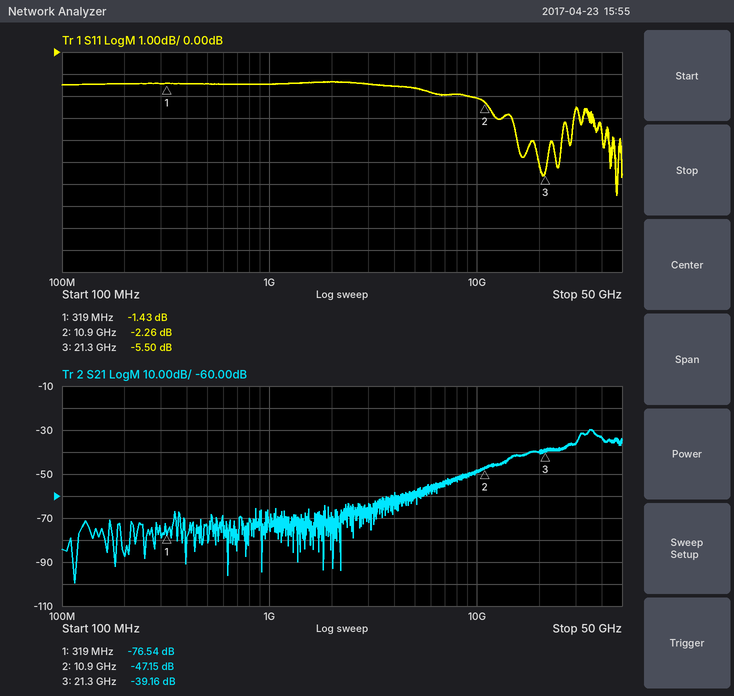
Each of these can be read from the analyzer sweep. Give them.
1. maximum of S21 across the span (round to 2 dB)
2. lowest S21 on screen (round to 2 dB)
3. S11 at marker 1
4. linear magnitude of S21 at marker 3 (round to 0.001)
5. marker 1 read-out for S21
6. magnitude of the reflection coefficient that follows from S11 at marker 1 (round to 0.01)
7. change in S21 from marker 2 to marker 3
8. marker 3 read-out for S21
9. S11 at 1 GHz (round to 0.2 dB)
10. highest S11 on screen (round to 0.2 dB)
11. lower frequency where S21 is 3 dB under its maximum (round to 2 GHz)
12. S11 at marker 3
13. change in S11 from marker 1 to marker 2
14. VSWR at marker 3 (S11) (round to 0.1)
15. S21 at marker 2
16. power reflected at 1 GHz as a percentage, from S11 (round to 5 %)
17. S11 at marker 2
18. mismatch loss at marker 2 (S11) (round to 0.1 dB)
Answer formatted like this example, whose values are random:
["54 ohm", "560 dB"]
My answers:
["-30 dB", "-100 dB", "-1.43 dB", "0.011", "-76.54 dB", "0.85", "7.99 dB", "-39.16 dB", "-1.4 dB", "-1.4 dB", "32 GHz", "-5.50 dB", "-0.83 dB", "3.3", "-47.15 dB", "70 %", "-2.26 dB", "3.9 dB"]
